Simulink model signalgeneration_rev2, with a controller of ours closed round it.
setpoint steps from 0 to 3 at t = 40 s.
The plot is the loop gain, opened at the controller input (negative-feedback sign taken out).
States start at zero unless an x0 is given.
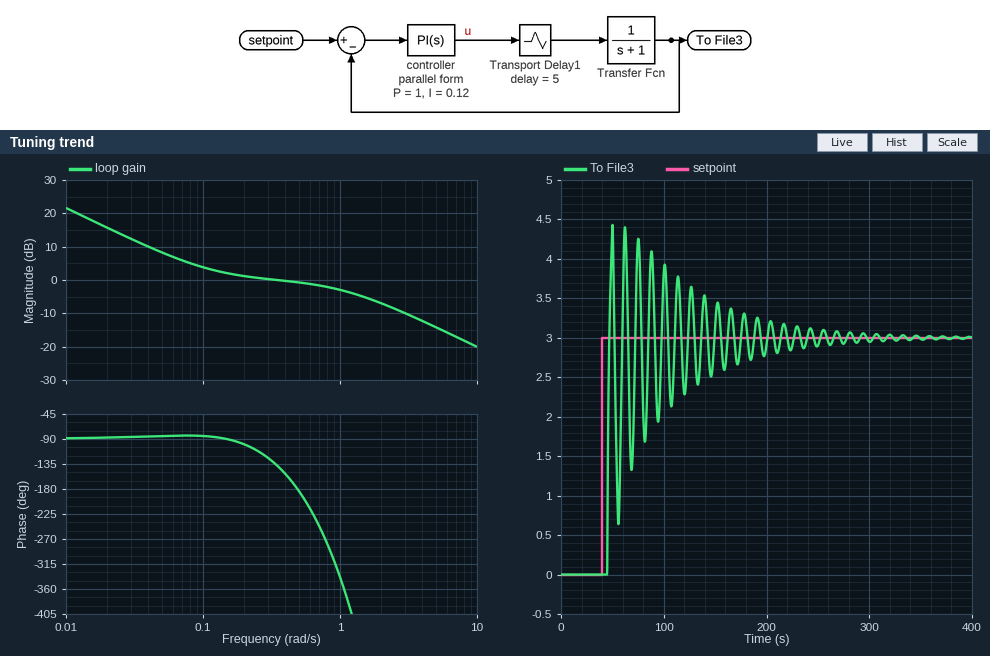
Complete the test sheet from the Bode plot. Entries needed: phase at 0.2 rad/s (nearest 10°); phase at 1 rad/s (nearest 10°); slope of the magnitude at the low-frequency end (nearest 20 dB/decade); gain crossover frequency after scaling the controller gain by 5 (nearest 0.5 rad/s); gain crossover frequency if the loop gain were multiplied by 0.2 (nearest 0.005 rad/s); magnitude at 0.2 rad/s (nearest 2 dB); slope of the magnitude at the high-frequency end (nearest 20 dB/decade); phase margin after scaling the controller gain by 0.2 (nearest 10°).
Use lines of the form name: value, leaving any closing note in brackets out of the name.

phase at 0.2 rad/s: -100°
phase at 1 rad/s: -340°
slope of the magnitude at the low-frequency end: -20 dB/decade
gain crossover frequency after scaling the controller gain by 5: 5.0 rad/s
gain crossover frequency if the loop gain were multiplied by 0.2: 0.025 rad/s
magnitude at 0.2 rad/s: 2 dB
slope of the magnitude at the high-frequency end: -20 dB/decade
phase margin after scaling the controller gain by 0.2: 90°
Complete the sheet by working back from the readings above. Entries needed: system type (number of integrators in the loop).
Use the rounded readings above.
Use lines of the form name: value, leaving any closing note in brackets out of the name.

system type: 1
